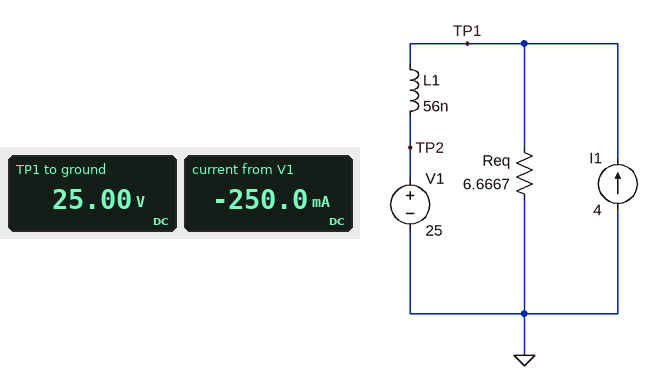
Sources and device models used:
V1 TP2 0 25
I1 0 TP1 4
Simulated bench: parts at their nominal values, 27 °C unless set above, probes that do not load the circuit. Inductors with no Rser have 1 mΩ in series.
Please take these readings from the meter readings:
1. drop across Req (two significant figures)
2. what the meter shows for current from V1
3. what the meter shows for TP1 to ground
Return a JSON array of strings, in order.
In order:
["25 V", "-250.0 mA", "25.00 V"]
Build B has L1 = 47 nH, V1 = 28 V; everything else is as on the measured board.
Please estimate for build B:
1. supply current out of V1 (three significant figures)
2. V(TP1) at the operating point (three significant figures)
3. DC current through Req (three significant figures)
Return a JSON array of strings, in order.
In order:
["200 mA", "28.0 V", "4.20 A"]
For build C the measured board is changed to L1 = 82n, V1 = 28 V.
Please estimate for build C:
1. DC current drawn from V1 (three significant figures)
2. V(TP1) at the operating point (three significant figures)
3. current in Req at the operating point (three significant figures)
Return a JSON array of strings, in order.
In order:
["200 mA", "28.0 V", "4.20 A"]
